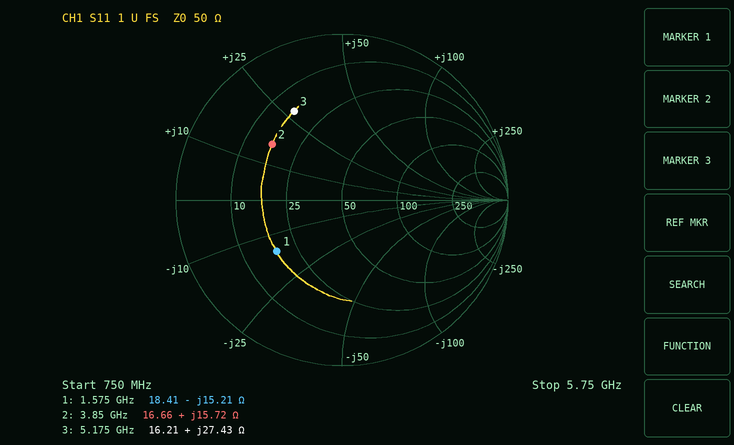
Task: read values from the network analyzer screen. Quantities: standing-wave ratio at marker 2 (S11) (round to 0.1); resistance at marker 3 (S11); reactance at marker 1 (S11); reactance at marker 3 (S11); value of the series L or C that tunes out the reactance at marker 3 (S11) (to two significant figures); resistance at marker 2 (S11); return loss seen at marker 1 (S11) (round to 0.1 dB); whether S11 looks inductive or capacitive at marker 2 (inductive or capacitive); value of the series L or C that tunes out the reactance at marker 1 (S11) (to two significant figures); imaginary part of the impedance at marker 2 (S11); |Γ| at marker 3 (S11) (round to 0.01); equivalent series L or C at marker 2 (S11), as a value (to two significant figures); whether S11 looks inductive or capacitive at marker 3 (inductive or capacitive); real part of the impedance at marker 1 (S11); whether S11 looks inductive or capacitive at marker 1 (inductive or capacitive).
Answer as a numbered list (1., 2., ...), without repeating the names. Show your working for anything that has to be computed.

1. 3.3
2. 16.21 Ω
3. -15.21 Ω
4. +27.43 Ω
5. C = 1/(2π × 5.175 GHz × 27.43 Ω) ≈ 1.1 pF
6. 16.66 Ω
7. 6.0 dB
8. inductive
9. L = 15.21 Ω/(2π × 1.575 GHz) ≈ 1.5 nH
10. +15.72 Ω
11. 0.61
12. L = 15.72 Ω/(2π × 3.85 GHz) ≈ 650 pH
13. inductive
14. 18.41 Ω
15. capacitive
